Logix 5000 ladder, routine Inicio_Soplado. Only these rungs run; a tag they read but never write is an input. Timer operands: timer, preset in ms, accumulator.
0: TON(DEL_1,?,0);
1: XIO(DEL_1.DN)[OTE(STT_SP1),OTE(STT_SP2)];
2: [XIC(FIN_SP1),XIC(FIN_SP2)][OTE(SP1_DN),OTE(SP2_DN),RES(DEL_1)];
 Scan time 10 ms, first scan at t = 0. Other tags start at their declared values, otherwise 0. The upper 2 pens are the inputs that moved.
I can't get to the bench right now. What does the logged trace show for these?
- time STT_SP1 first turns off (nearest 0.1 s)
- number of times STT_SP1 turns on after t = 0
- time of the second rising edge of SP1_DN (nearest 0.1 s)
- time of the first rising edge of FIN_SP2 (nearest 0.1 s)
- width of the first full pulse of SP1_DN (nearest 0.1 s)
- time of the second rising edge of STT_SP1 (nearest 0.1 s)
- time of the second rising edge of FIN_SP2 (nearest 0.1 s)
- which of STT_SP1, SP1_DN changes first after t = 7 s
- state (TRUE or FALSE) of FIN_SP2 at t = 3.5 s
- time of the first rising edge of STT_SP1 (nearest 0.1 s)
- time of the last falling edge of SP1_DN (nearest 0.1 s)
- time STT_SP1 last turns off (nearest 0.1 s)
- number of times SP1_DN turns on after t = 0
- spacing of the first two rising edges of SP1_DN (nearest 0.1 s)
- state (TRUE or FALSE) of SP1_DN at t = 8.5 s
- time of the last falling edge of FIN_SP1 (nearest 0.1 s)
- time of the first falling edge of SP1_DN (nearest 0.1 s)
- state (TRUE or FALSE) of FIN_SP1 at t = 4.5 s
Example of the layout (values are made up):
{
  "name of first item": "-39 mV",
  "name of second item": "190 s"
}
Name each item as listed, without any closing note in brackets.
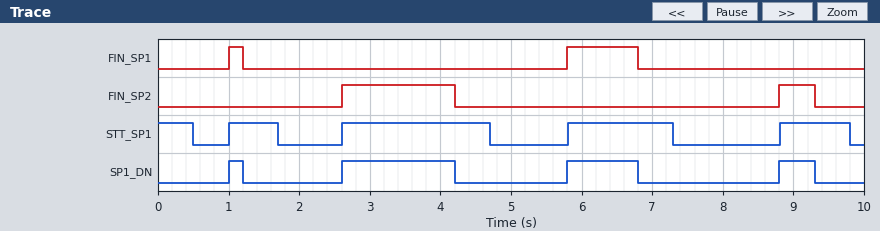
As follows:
{
  "time STT_SP1 first turns off": "0.5 s",
  "number of times STT_SP1 turns on after t = 0": "4",
  "time of the second rising edge of SP1_DN": "2.6 s",
  "time of the first rising edge of FIN_SP2": "2.6 s",
  "width of the first full pulse of SP1_DN": "0.2 s",
  "time of the second rising edge of STT_SP1": "2.6 s",
  "time of the second rising edge of FIN_SP2": "8.8 s",
  "which of STT_SP1, SP1_DN changes first after t = 7 s": "STT_SP1",
  "state (TRUE or FALSE) of FIN_SP2 at t = 3.5 s": "TRUE",
  "time of the first rising edge of STT_SP1": "1.0 s",
  "time of the last falling edge of SP1_DN": "9.3 s",
  "time STT_SP1 last turns off": "9.8 s",
  "number of times SP1_DN turns on after t = 0": "4",
  "spacing of the first two rising edges of SP1_DN": "1.6 s",
  "state (TRUE or FALSE) of SP1_DN at t = 8.5 s": "FALSE",
  "time of the last falling edge of FIN_SP1": "6.8 s",
  "time of the first falling edge of SP1_DN": "1.2 s",
  "state (TRUE or FALSE) of FIN_SP1 at t = 4.5 s": "FALSE"
}
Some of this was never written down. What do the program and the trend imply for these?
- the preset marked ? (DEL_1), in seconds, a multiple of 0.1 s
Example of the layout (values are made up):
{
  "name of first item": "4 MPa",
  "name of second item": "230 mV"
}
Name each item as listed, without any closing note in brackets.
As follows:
{
  "the preset marked ? (DEL_1), in seconds, a multiple of 0.1 s": "0.5 s"
}
